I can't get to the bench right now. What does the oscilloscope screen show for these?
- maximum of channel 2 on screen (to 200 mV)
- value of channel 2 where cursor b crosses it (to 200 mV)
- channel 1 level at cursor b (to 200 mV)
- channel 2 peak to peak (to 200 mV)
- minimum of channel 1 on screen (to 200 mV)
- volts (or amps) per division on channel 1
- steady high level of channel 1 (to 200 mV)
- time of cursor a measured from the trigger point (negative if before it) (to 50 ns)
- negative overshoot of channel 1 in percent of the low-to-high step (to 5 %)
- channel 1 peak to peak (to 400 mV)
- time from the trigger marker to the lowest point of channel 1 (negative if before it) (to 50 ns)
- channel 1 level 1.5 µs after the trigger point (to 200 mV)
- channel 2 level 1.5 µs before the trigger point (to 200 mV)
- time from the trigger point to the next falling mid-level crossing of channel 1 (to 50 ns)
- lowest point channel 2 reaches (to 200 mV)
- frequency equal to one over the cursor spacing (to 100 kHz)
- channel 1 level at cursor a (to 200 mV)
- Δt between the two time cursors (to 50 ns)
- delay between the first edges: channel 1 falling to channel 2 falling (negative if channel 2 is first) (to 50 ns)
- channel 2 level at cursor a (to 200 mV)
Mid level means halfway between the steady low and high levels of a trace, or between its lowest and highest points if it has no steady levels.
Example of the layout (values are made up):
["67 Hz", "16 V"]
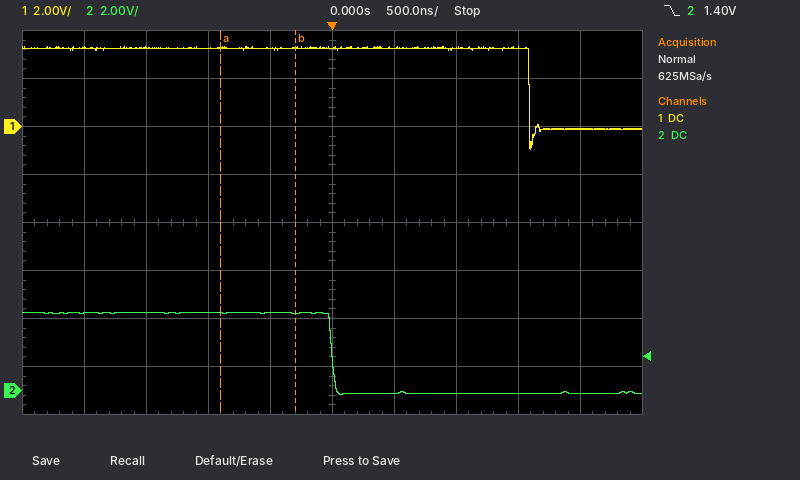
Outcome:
["3.2 V", "3.2 V", "3.2 V", "3.4 V", "-1.0 V", "2 V", "3.2 V", "-900 ns", "25 %", "4.4 V", "+1.60 µs", "3.2 V", "3.2 V", "1.60 µs", "-200 mV", "1.7 MHz", "3.2 V", "600 ns", "-1.60 µs", "3.2 V"]
